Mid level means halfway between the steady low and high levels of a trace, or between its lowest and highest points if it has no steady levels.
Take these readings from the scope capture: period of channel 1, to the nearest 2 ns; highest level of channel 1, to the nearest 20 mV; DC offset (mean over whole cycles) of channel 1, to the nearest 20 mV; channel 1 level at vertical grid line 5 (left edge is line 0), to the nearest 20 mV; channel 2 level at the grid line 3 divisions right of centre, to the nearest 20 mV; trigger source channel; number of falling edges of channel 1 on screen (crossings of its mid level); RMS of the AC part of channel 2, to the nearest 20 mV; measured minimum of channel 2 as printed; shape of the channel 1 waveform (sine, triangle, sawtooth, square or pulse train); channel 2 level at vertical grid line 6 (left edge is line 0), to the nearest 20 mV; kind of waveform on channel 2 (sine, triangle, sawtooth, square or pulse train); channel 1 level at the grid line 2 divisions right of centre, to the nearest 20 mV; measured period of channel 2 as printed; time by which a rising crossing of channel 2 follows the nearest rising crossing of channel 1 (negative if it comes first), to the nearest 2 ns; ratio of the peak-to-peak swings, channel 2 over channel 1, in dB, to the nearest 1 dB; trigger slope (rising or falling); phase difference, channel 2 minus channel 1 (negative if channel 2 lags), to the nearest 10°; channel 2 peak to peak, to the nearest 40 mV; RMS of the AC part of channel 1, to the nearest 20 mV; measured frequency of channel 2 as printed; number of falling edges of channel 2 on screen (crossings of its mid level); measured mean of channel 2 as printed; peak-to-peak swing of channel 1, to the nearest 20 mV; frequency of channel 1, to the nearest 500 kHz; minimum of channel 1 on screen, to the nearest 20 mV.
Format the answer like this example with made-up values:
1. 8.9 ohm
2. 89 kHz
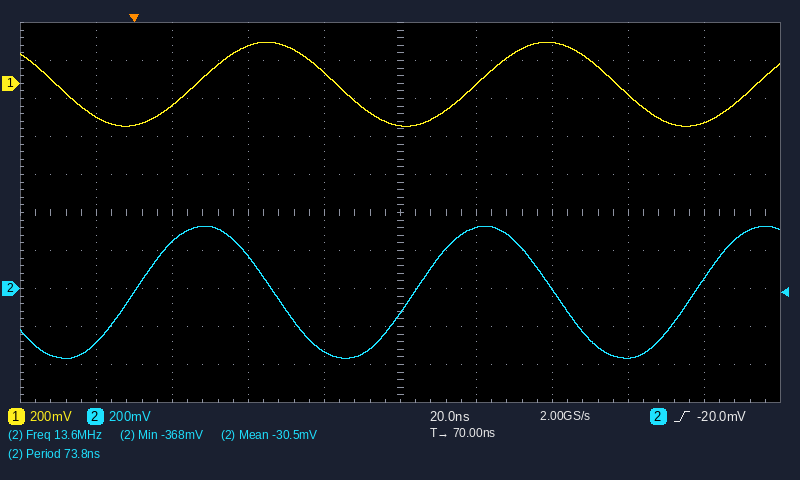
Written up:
1. 74 ns
2. 220 mV
3. 0 mV
4. -220 mV
5. -360 mV
6. channel 2
7. 3
8. 240 mV
9. -368 mV
10. sine
11. 320 mV
12. sine
13. 220 mV
14. 73.8 ns
15. -16 ns
16. 4 dB
17. rising
18. +80°
19. 680 mV
20. 160 mV
21. 13.6 MHz
22. 2
23. -30.5 mV
24. 440 mV
25. 13.5 MHz
26. -220 mV
